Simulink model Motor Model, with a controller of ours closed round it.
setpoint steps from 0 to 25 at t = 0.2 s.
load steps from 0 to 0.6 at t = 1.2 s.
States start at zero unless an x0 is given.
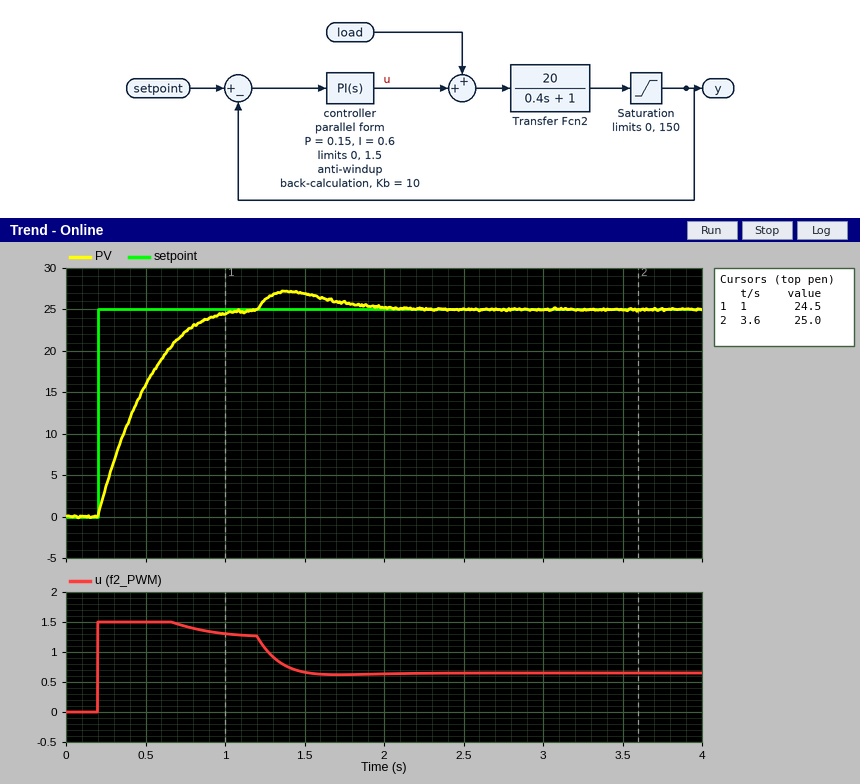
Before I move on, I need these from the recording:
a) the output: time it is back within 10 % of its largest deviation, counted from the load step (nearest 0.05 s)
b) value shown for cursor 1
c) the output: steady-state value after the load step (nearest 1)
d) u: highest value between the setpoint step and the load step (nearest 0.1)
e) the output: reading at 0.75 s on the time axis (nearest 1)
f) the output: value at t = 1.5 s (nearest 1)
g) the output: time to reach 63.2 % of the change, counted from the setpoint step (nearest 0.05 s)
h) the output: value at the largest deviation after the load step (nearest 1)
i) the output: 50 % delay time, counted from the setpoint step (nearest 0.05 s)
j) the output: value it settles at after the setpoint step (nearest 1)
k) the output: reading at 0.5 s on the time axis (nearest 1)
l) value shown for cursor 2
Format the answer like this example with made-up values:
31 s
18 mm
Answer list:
0.80 s
24.5
25
1.5
22
27
0.30 s
27
0.20 s
25
16
25.0
